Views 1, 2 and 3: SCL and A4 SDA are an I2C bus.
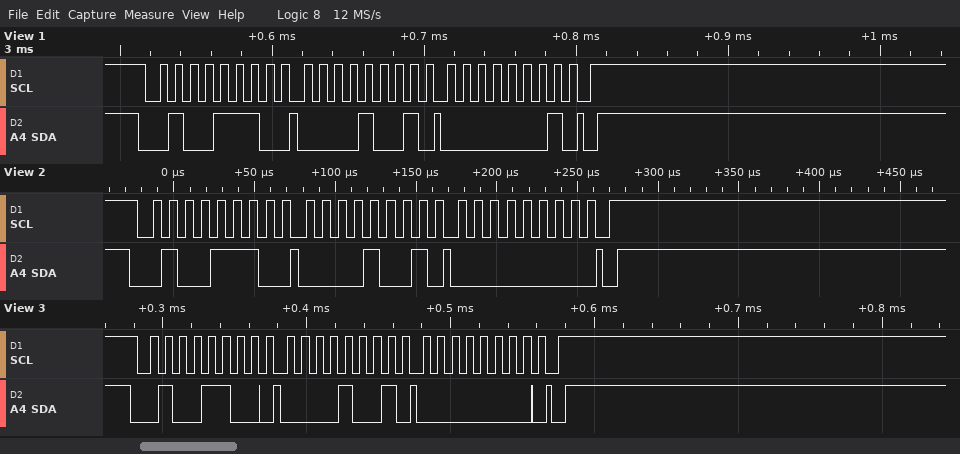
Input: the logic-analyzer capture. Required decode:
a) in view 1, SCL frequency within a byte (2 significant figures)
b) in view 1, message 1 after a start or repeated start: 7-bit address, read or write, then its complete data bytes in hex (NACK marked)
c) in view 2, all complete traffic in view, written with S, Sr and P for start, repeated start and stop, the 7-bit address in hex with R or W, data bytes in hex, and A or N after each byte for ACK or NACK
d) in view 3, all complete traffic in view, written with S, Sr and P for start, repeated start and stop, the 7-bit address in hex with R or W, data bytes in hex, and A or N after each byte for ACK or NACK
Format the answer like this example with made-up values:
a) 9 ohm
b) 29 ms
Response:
a) 100 kHz
b) 0x27 write: 09 01
c) S 27W A 09 A 00 A P
d) S 26W A 09 A 00 A P
